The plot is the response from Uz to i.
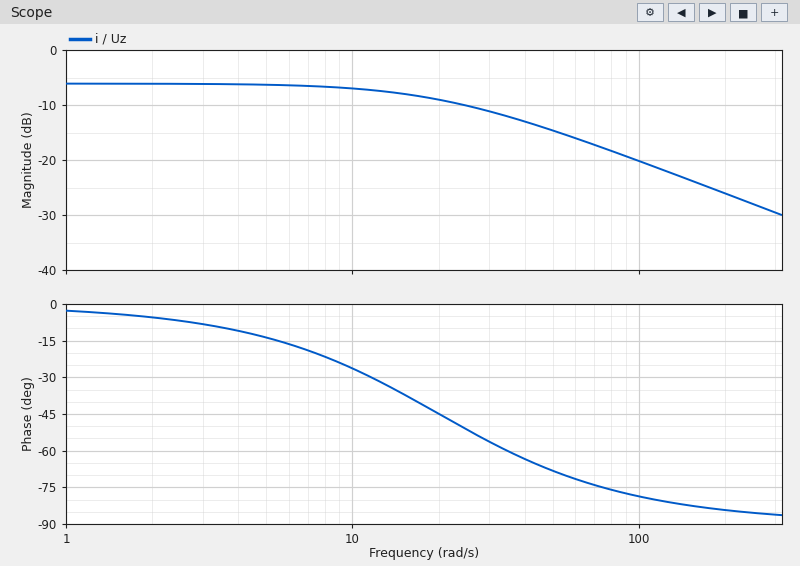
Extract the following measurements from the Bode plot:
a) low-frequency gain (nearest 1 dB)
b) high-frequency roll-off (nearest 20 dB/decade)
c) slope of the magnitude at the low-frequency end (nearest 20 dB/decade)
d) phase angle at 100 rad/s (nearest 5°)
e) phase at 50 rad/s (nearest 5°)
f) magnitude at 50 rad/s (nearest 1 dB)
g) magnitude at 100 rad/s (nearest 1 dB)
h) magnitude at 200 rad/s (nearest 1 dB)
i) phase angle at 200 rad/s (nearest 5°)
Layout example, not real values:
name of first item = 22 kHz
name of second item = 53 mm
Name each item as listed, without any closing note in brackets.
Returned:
low-frequency gain = -6 dB
high-frequency roll-off = -20 dB/decade
slope of the magnitude at the low-frequency end = 0 dB/decade
phase angle at 100 rad/s = -80°
phase at 50 rad/s = -70°
magnitude at 50 rad/s = -15 dB
magnitude at 100 rad/s = -20 dB
magnitude at 200 rad/s = -26 dB
phase angle at 200 rad/s = -85°
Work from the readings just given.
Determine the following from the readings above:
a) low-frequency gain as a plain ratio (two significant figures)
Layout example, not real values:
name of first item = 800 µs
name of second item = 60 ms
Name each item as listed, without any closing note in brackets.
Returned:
low-frequency gain as a plain ratio = 0.50
